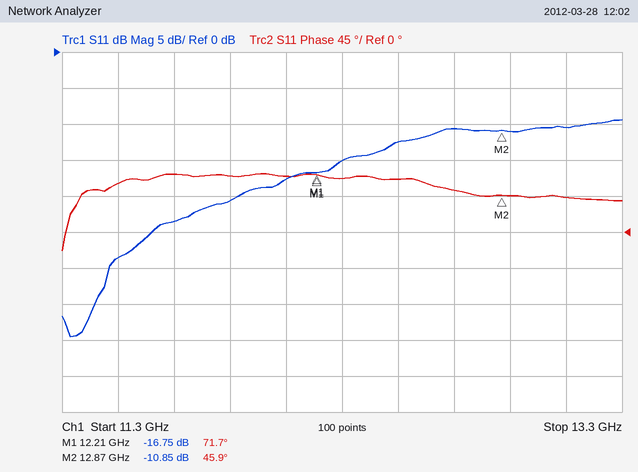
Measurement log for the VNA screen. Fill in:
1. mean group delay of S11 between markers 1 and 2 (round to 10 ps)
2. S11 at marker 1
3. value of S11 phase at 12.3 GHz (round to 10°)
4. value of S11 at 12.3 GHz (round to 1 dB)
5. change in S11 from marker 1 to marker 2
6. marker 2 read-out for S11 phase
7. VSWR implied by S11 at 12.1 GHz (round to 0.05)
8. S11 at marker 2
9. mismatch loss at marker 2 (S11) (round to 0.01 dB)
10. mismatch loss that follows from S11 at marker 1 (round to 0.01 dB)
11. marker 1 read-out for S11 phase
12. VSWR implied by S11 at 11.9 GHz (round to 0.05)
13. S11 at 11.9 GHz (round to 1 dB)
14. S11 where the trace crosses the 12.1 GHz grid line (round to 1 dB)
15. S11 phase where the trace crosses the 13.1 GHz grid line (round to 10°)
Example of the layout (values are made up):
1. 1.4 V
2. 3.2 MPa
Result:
1. 110 ps
2. -16.75 dB
3. 70°
4. -15 dB
5. 5.90 dB
6. 45.9°
7. 1.30
8. -10.85 dB
9. 0.37 dB
10. 0.09 dB
11. 71.7°
12. 1.20
13. -21 dB
14. -18 dB
15. 40°
